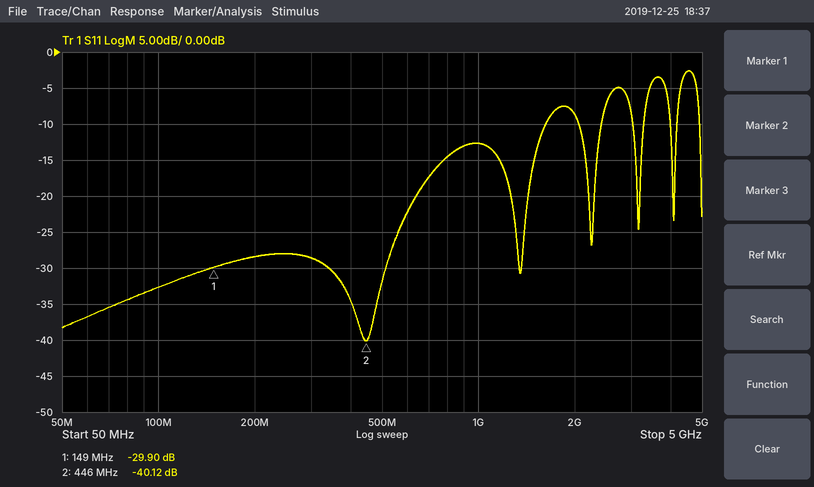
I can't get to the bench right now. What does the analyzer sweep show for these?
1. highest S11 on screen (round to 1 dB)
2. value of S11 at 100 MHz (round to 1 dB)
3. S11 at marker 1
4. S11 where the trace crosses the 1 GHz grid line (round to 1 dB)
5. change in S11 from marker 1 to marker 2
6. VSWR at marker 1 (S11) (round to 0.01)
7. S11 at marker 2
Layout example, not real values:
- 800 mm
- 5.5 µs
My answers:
- -3 dB
- -33 dB
- -29.90 dB
- -13 dB
- -10.22 dB
- 1.07
- -40.12 dB
